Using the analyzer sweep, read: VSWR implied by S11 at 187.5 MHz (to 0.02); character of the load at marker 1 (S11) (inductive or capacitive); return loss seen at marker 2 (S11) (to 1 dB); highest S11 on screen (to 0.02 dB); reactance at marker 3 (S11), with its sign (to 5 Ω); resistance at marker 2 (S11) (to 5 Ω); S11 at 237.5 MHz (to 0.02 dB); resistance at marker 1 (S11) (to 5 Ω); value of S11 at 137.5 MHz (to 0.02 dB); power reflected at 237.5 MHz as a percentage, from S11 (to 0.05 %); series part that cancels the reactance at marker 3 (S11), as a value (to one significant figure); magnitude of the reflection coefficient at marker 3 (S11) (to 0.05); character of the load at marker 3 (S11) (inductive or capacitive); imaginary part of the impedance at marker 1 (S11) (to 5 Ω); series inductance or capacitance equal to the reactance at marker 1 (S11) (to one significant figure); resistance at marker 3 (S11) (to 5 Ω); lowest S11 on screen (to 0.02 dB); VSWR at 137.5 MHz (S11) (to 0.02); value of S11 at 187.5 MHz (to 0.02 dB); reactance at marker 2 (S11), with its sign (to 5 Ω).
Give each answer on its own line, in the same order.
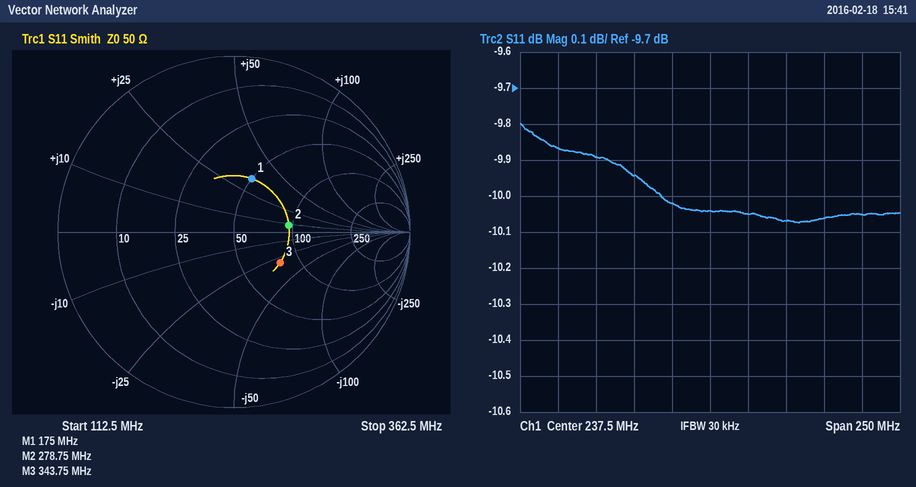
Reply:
1.94
inductive
10 dB
-9.80 dB
-30 Ω
95 Ω
-10.04 dB
50 Ω
-9.86 dB
9.90 %
10 nH
0.30
capacitive
+35 Ω
30 nH
80 Ω
-10.08 dB
1.94
-9.94 dB
+10 Ω
